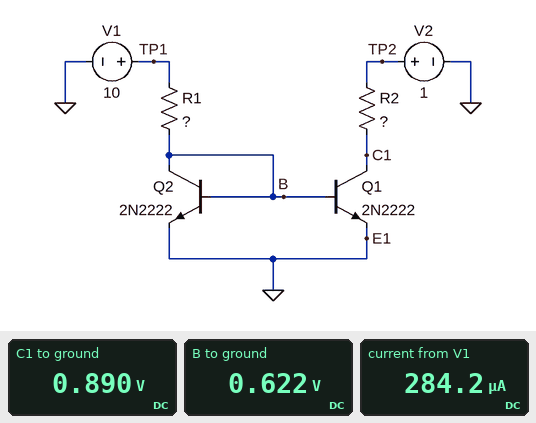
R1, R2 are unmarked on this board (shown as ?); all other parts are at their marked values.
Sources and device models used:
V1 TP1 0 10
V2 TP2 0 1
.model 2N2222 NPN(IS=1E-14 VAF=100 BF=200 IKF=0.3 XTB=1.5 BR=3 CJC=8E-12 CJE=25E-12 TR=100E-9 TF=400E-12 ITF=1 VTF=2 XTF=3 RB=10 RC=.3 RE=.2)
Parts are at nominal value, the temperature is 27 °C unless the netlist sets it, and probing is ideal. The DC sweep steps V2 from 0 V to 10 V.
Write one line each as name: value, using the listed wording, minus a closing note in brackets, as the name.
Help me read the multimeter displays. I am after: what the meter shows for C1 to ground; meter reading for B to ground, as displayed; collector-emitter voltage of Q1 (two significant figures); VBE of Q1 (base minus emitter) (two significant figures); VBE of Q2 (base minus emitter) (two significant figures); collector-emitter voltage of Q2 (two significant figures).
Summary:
what the meter shows for C1 to ground: 0.890 V
meter reading for B to ground, as displayed: 0.622 V
collector-emitter voltage of Q1: 890 mV
VBE of Q1 (base minus emitter): 620 mV
VBE of Q2 (base minus emitter): 620 mV
collector-emitter voltage of Q2: 620 mV
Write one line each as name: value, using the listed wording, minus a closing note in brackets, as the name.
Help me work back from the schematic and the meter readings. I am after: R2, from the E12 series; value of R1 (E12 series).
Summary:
R2, from the E12 series: 390 Ω
value of R1: 33 kΩ
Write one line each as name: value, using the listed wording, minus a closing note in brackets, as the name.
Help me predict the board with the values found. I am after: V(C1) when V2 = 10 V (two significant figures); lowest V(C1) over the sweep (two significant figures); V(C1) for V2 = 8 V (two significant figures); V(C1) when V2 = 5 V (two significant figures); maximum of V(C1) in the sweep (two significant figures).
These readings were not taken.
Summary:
V(C1) when V2 = 10 V: 9.9 V
lowest V(C1) over the sweep: 5.8 mV
V(C1) for V2 = 8 V: 7.9 V
V(C1) when V2 = 5 V: 4.9 V
maximum of V(C1) in the sweep: 9.9 V
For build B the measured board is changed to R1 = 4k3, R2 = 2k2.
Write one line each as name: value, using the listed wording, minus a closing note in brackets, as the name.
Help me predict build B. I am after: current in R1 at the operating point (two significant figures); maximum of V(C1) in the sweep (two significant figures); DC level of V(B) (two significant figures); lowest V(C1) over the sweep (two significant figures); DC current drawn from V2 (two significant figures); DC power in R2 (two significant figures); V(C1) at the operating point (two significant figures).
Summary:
current in R1 at the operating point: 2.2 mA
maximum of V(C1) in the sweep: 5.1 V
DC level of V(B): 670 mV
lowest V(C1) over the sweep: 7.5 mV
DC current drawn from V2: 450 µA
DC power in R2: 440 µW
V(C1) at the operating point: 16 mV
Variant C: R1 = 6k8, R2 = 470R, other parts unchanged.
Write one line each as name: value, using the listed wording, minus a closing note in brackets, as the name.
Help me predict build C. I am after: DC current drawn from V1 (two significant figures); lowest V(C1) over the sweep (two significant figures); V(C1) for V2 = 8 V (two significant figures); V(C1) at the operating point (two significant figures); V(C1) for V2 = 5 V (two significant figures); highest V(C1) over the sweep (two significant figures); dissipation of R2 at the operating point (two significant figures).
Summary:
DC current drawn from V1: 1.4 mA
lowest V(C1) over the sweep: 7.2 mV
V(C1) for V2 = 8 V: 7.3 V
V(C1) at the operating point: 360 mV
V(C1) for V2 = 5 V: 4.3 V
highest V(C1) over the sweep: 9.3 V
dissipation of R2 at the operating point: 860 µW
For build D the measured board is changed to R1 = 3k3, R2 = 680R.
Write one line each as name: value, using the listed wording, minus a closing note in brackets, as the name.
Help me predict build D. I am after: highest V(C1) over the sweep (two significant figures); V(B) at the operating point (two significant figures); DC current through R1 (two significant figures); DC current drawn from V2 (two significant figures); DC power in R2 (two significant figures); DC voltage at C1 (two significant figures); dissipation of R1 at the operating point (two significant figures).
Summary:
highest V(C1) over the sweep: 8.0 V
V(B) at the operating point: 680 mV
DC current through R1: 2.8 mA
DC current drawn from V2: 1.4 mA
DC power in R2: 1.4 mW
DC voltage at C1: 32 mV
dissipation of R1 at the operating point: 26 mW
